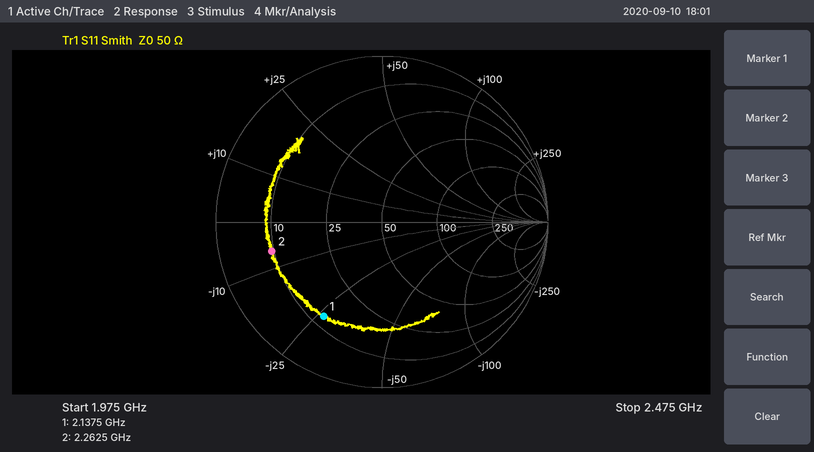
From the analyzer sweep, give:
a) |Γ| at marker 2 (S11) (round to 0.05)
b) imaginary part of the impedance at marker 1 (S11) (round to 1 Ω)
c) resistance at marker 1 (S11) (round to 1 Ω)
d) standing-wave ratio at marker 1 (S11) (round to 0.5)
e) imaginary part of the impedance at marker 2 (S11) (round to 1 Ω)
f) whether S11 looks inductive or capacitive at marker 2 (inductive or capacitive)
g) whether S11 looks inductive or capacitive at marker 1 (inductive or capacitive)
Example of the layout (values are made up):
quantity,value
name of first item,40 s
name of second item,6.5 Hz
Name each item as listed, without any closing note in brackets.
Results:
quantity,value
|Γ| at marker 2 (S11),0.70
imaginary part of the impedance at marker 1 (S11),-26 Ω
resistance at marker 1 (S11),13 Ω
standing-wave ratio at marker 1 (S11),5.0
imaginary part of the impedance at marker 2 (S11),-6 Ω
whether S11 looks inductive or capacitive at marker 2,capacitive
whether S11 looks inductive or capacitive at marker 1,capacitive
